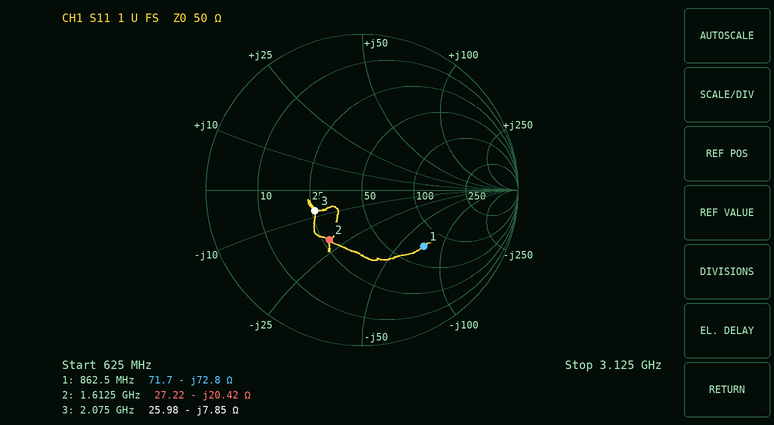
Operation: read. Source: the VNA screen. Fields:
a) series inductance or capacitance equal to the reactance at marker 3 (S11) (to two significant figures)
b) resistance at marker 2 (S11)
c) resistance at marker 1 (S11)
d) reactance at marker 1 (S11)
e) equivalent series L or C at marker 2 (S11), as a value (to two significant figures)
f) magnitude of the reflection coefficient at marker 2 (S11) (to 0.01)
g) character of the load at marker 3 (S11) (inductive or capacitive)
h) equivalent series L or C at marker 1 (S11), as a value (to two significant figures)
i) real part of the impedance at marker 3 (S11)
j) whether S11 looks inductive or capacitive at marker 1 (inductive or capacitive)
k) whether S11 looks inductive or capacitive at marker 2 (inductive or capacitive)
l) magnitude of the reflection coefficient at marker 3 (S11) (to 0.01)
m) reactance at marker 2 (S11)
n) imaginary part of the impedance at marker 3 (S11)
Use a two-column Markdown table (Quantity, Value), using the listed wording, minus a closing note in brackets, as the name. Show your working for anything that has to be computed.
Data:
| Quantity | Value |
|---|---|
| series inductance or capacitance equal to the reactance at marker 3 (S11) | C = 1/(2π × 2.075 GHz × 7.85 Ω) ≈ 9.8 pF |
| resistance at marker 2 | 27.22 Ω |
| resistance at marker 1 | 71.7 Ω |
| reactance at marker 1 | -72.8 Ω |
| equivalent series L or C at marker 2 (S11), as a value | C = 1/(2π × 1.6125 GHz × 20.42 Ω) ≈ 4.8 pF |
| magnitude of the reflection coefficient at marker 2 (S11) | 0.38 |
| character of the load at marker 3 (S11) | capacitive |
| equivalent series L or C at marker 1 (S11), as a value | C = 1/(2π × 862.5 MHz × 72.8 Ω) ≈ 2.5 pF |
| real part of the impedance at marker 3 | 25.98 Ω |
| whether S11 looks inductive or capacitive at marker 1 | capacitive |
| whether S11 looks inductive or capacitive at marker 2 | capacitive |
| magnitude of the reflection coefficient at marker 3 (S11) | 0.33 |
| reactance at marker 2 | -20.42 Ω |
| imaginary part of the impedance at marker 3 | -7.85 Ω |
